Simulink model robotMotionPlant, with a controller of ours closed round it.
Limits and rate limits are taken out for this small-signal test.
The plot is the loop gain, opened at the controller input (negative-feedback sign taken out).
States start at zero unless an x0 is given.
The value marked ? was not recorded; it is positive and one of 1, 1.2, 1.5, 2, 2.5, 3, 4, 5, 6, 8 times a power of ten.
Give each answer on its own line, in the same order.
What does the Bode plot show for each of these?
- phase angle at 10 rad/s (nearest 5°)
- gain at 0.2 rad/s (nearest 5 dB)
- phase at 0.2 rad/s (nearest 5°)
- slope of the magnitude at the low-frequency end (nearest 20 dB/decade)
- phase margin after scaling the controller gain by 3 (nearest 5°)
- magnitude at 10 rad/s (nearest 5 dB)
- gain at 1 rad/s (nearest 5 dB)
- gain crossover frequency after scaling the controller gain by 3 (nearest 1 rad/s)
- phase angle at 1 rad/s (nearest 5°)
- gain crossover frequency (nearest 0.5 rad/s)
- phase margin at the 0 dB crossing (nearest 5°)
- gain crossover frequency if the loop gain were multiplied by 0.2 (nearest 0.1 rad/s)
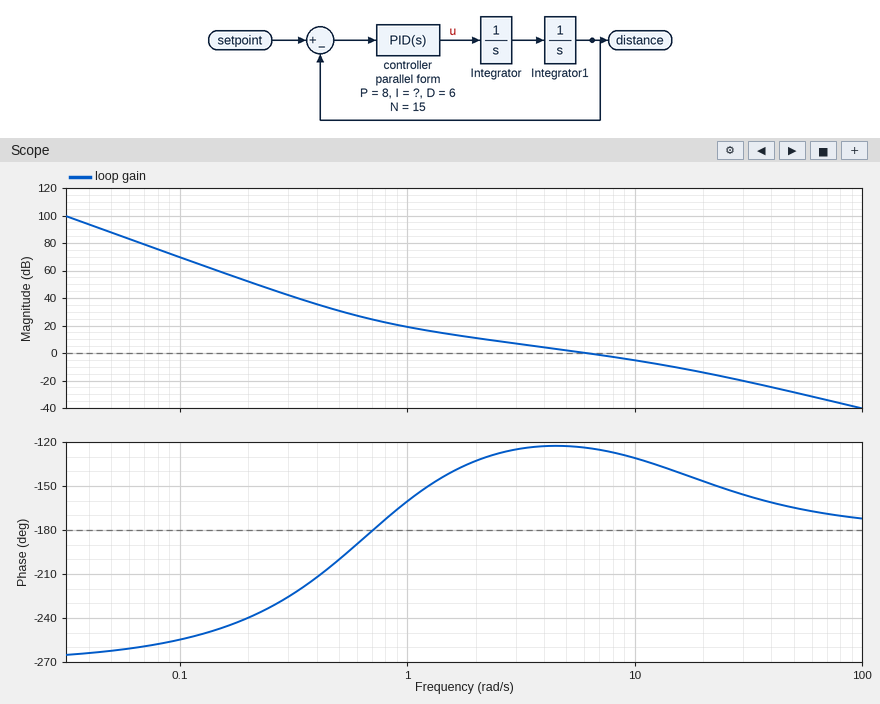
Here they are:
-130°
50 dB
-240°
-60 dB/decade
40°
-5 dB
20 dB
14 rad/s
-160°
6.0 rad/s
55°
1.5 rad/s
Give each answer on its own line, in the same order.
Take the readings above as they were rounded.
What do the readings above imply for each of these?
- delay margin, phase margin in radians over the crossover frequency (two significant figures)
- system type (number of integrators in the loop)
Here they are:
0.16 s
3
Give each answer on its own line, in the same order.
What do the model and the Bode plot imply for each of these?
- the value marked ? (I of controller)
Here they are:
3
